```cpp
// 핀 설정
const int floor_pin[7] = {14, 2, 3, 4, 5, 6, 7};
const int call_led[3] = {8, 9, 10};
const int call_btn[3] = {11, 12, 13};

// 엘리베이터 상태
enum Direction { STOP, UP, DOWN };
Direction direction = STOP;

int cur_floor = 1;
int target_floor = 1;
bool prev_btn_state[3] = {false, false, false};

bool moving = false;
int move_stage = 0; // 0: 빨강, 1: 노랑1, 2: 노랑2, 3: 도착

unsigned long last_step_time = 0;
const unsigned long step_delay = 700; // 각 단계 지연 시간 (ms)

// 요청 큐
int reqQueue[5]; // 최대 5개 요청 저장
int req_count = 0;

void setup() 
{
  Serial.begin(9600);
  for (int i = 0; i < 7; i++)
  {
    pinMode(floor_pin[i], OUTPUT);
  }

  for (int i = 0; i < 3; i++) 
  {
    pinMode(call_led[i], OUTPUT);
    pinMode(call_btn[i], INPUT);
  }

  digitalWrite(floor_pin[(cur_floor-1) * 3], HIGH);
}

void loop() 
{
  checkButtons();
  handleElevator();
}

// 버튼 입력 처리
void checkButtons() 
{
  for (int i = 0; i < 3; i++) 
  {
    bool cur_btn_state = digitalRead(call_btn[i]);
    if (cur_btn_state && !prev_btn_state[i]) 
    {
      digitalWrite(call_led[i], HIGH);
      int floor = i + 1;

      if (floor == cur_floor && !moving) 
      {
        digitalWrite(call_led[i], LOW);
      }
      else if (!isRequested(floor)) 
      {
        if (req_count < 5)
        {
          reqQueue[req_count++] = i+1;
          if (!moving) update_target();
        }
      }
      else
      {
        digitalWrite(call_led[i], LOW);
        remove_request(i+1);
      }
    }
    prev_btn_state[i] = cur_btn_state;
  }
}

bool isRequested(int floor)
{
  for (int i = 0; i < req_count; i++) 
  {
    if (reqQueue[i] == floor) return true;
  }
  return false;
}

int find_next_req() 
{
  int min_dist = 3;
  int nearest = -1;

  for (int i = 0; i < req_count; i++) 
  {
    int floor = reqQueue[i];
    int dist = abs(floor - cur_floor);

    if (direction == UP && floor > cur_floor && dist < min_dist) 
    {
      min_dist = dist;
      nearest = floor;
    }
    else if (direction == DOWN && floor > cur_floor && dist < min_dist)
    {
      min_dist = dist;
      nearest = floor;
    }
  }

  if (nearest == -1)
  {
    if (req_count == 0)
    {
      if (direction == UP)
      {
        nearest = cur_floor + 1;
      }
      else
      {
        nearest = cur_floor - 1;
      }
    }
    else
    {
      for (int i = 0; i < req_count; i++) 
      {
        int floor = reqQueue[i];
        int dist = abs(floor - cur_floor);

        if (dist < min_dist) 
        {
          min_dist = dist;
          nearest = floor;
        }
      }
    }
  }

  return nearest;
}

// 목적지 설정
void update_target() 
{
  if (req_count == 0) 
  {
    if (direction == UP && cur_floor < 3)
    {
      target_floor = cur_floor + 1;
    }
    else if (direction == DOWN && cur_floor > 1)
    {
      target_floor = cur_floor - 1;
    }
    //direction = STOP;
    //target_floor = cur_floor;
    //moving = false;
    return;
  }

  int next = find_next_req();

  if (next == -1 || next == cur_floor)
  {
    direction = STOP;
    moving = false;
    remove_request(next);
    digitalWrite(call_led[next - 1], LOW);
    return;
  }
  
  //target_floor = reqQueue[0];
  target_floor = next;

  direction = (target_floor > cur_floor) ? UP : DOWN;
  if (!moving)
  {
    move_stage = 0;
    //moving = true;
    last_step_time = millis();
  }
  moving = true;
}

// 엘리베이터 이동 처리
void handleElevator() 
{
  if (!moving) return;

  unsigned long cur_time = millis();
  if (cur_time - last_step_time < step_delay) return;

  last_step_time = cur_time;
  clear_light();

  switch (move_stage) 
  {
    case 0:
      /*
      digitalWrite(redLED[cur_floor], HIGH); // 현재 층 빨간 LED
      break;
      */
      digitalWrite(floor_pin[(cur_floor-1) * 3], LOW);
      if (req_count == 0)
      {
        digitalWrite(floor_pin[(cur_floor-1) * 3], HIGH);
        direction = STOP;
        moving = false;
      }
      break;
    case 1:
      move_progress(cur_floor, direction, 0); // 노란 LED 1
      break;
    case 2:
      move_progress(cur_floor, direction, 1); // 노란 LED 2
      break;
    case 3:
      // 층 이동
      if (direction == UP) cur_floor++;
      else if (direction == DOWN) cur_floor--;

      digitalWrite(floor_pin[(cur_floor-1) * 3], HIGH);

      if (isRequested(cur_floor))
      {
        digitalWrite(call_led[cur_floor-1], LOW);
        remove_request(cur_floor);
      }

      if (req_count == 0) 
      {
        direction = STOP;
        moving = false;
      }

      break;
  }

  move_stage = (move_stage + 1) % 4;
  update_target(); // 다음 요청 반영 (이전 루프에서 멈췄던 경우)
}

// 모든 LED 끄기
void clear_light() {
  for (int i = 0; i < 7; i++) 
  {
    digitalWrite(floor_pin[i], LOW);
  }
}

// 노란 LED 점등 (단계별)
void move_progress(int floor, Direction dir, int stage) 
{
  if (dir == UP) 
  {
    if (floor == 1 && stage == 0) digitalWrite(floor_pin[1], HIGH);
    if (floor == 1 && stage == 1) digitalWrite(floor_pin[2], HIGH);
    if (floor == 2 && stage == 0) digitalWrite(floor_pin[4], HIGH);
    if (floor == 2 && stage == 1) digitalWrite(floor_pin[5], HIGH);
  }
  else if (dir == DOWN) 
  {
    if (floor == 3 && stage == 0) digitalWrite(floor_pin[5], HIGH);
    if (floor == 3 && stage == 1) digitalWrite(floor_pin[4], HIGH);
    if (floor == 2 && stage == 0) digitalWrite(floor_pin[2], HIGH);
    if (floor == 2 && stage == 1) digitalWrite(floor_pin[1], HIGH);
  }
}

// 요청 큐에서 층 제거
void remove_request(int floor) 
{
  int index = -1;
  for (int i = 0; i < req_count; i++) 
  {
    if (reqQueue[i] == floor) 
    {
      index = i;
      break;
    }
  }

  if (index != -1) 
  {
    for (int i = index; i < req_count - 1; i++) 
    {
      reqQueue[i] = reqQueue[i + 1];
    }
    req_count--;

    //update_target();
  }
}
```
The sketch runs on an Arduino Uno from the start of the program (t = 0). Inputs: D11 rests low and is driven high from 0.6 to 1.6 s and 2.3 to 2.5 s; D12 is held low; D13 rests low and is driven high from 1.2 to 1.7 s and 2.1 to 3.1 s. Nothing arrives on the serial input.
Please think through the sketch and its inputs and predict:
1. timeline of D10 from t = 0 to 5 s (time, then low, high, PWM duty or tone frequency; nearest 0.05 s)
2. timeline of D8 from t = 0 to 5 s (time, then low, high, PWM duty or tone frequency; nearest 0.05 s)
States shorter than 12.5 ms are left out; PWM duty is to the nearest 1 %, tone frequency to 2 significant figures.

0 s low; 1.2 s high; 2.1 s low
0 s low; 2.3 s high; 2.6 s low
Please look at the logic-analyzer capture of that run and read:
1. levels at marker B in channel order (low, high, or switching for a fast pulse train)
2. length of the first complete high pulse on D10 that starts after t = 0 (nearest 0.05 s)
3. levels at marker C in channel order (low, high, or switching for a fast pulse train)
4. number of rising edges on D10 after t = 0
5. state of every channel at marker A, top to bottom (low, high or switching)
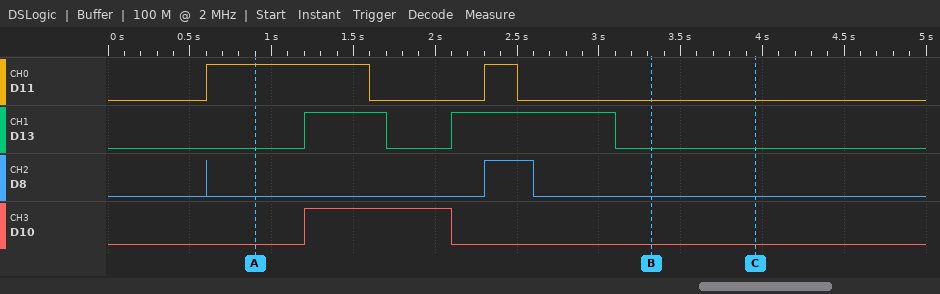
D11 low, D13 low, D8 low, D10 low
0.90 s
D11 low, D13 low, D8 low, D10 low
1
D11 high, D13 low, D8 low, D10 low
